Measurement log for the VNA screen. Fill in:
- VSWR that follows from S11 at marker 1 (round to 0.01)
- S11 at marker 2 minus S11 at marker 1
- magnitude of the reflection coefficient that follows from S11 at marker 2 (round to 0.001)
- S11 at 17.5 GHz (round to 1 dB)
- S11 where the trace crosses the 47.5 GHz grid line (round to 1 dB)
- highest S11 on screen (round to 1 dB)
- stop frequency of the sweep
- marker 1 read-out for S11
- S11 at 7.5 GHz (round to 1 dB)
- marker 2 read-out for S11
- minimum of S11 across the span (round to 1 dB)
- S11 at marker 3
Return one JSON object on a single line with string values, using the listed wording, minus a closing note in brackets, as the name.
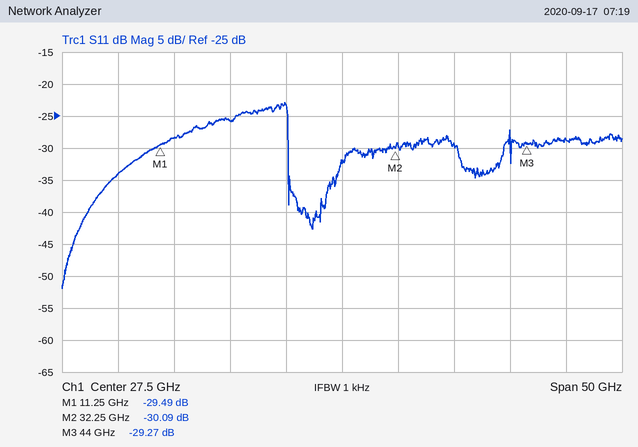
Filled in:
{"VSWR that follows from S11 at marker 1": "1.07", "S11 at marker 2 minus S11 at marker 1": "-0.60 dB", "magnitude of the reflection coefficient that follows from S11 at marker 2": "0.031", "S11 at 17.5 GHz": "-26 dB", "S11 where the trace crosses the 47.5 GHz grid line": "-29 dB", "highest S11 on screen": "-23 dB", "stop frequency of the sweep": "52.5 GHz", "marker 1 read-out for S11": "-29.49 dB", "S11 at 7.5 GHz": "-34 dB", "marker 2 read-out for S11": "-30.09 dB", "minimum of S11 across the span": "-52 dB", "S11 at marker 3": "-29.27 dB"}
